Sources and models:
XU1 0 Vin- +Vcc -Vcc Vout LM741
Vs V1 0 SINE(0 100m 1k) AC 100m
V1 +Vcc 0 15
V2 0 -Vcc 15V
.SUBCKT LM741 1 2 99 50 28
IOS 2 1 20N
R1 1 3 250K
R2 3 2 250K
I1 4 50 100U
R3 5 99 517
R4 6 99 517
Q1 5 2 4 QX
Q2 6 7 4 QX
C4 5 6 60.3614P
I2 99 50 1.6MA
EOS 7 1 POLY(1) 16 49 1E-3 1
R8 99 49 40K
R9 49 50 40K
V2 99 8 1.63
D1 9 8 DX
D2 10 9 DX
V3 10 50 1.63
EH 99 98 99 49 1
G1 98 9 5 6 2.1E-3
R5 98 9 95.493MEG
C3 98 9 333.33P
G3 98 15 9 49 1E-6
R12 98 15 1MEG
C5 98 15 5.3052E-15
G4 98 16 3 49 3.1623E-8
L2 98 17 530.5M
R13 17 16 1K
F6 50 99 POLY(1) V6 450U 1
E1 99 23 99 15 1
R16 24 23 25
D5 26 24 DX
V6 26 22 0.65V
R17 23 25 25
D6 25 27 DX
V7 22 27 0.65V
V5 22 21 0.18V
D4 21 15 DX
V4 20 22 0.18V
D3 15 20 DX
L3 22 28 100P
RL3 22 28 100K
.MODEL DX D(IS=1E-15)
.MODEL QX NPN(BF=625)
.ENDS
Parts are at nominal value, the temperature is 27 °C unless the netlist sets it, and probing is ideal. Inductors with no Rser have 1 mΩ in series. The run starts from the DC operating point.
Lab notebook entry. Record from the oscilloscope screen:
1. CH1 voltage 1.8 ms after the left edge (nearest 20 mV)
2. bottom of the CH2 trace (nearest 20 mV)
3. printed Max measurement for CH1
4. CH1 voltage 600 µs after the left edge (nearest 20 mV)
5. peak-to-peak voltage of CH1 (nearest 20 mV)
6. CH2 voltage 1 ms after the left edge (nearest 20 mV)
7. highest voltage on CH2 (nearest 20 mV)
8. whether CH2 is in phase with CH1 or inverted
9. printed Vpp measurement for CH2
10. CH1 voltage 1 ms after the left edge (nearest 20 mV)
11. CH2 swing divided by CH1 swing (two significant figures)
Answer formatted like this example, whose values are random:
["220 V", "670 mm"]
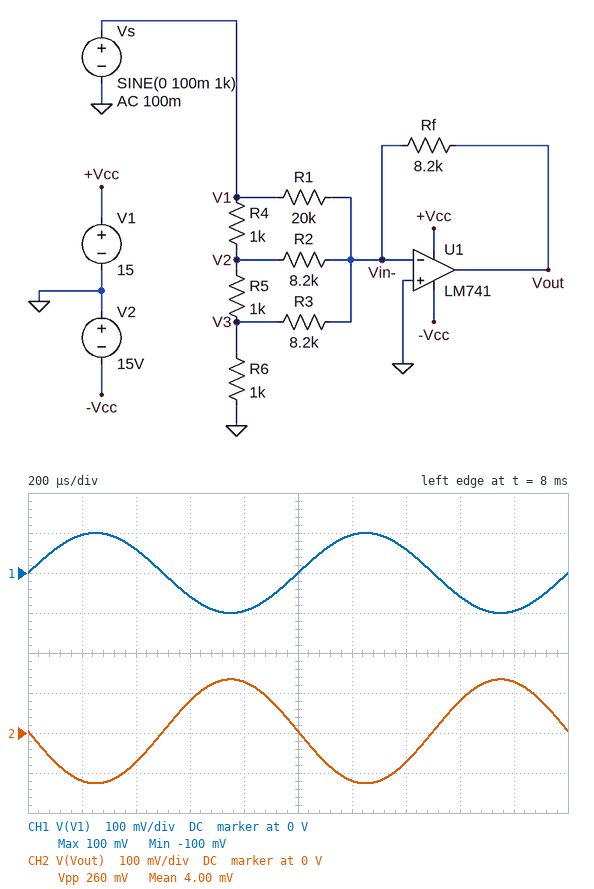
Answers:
["-100 mV", "-120 mV", "100 mV", "-60 mV", "200 mV", "0 V", "140 mV", "inverted", "260 mV", "0 V", "1.3"]
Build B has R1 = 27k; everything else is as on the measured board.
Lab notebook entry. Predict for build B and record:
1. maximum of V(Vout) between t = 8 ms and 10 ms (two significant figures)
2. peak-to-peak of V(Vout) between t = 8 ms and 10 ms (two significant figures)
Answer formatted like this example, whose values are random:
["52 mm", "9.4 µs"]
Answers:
["120 mV", "240 mV"]
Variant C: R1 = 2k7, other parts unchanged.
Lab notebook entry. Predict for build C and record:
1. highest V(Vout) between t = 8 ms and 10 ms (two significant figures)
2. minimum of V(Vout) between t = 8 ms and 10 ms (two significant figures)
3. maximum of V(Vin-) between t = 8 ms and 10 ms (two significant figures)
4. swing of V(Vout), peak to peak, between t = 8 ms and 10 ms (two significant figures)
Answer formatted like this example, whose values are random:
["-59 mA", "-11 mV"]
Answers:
["400 mV", "-390 mV", "1.4 mV", "790 mV"]
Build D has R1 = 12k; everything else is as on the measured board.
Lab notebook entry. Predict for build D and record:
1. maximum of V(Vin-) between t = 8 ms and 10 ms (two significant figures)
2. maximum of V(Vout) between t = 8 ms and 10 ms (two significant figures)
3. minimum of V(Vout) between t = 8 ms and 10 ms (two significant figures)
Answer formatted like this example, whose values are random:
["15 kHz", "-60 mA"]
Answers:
["1.2 mV", "160 mV", "-150 mV"]
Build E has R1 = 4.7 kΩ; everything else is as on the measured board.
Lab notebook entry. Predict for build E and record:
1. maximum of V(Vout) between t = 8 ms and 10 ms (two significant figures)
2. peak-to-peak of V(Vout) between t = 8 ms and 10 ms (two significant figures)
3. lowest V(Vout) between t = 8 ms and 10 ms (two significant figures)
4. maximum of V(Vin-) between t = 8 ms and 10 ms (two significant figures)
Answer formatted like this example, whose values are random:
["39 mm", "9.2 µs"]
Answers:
["270 mV", "530 mV", "-260 mV", "1.3 mV"]
